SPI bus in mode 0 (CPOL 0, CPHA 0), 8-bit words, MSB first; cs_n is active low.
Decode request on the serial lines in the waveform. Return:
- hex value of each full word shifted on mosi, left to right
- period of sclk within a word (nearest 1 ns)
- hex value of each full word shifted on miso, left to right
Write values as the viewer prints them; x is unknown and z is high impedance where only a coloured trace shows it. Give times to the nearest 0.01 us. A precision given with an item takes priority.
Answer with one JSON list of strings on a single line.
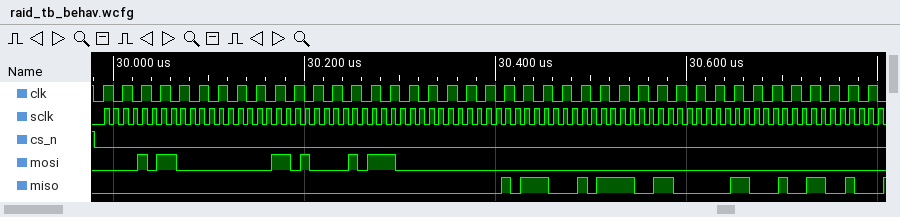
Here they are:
["0B, 00, 34, 2E, 00, 00, 00, 00, 00, 00", "10 ns", "00, 00, 00, 00, 00, 2E, 2F, 30, 31, 32"]
